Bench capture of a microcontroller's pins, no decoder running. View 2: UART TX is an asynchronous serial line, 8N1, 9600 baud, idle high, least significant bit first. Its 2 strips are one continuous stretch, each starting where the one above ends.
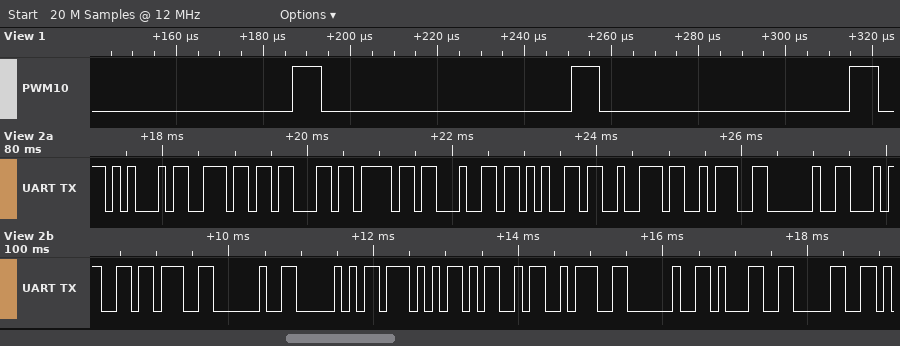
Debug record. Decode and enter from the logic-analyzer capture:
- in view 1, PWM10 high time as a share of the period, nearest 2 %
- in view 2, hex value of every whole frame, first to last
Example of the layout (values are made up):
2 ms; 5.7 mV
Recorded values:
10 %; 45 6E 63 6F 64 65 72 3A 20 34 3B 20 50 57 4D 3A 20 31 30
